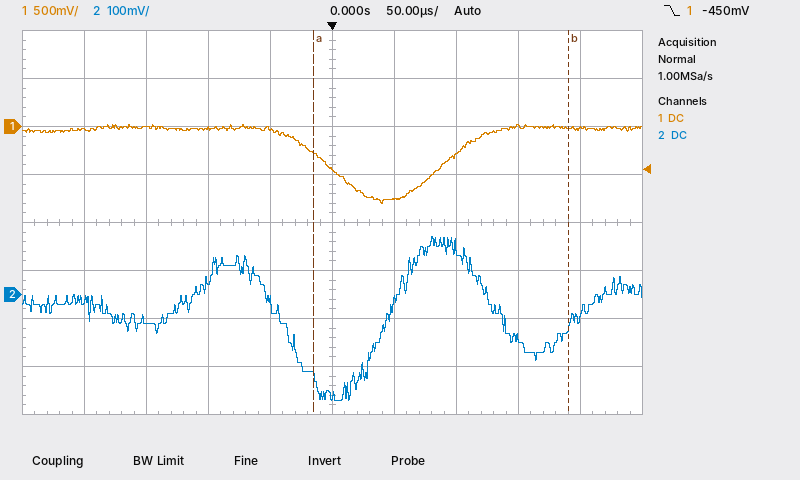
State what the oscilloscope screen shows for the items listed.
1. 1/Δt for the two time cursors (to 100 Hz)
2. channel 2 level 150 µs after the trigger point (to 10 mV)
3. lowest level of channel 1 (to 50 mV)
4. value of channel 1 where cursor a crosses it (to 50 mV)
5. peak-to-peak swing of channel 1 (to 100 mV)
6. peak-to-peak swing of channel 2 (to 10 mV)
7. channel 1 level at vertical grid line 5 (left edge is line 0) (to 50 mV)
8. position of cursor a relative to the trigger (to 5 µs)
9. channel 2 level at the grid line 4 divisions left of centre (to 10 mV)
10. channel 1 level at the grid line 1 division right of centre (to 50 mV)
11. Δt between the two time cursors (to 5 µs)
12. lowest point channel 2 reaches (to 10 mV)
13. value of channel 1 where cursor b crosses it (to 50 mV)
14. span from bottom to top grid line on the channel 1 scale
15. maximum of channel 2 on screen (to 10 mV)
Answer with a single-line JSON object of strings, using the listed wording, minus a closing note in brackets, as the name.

{"1/Δt for the two time cursors": "4.9 kHz", "channel 2 level 150 µs after the trigger point": "-90 mV", "lowest level of channel 1": "-800 mV", "value of channel 1 where cursor a crosses it": "-300 mV", "peak-to-peak swing of channel 1": "800 mV", "peak-to-peak swing of channel 2": "340 mV", "channel 1 level at vertical grid line 5 (left edge is line 0)": "-450 mV", "position of cursor a relative to the trigger": "-15 µs", "channel 2 level at the grid line 4 divisions left of centre": "-10 mV", "channel 1 level at the grid line 1 division right of centre": "-750 mV", "Δt between the two time cursors": "205 µs", "lowest point channel 2 reaches": "-220 mV", "value of channel 1 where cursor b crosses it": "0 mV", "span from bottom to top grid line on the channel 1 scale": "4 V", "maximum of channel 2 on screen": "120 mV"}
